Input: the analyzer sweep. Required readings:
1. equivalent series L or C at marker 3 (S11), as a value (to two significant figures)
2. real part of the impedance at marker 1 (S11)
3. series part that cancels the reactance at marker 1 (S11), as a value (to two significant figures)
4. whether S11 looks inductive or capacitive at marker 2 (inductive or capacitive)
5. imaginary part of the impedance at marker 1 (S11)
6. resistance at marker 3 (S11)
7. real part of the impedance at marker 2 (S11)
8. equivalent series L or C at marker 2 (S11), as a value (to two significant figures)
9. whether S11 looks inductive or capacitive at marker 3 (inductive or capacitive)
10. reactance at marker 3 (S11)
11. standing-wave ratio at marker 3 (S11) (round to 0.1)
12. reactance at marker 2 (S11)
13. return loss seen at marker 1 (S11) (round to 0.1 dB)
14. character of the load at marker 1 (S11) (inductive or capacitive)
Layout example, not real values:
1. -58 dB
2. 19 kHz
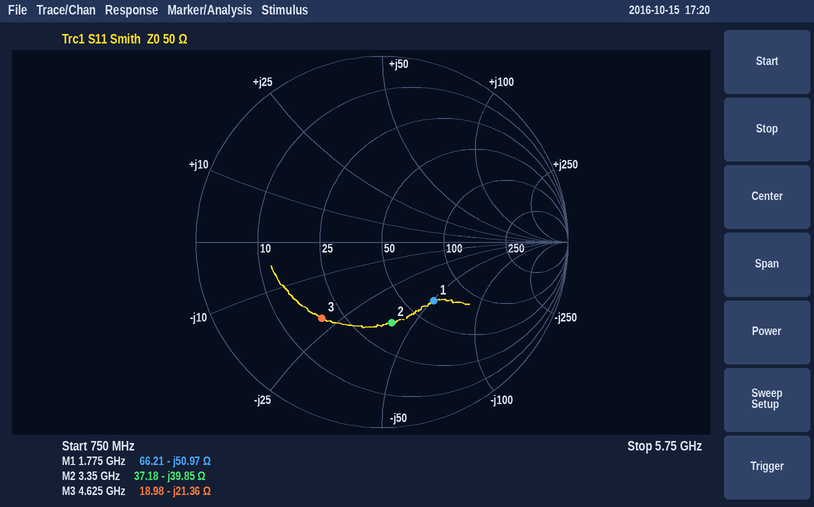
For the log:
1. 1.6 pF
2. 66.21 Ω
3. 4.6 nH
4. capacitive
5. -50.97 Ω
6. 18.98 Ω
7. 37.18 Ω
8. 1.2 pF
9. capacitive
10. -21.36 Ω
11. 3.2
12. -39.85 Ω
13. 7.5 dB
14. capacitive
